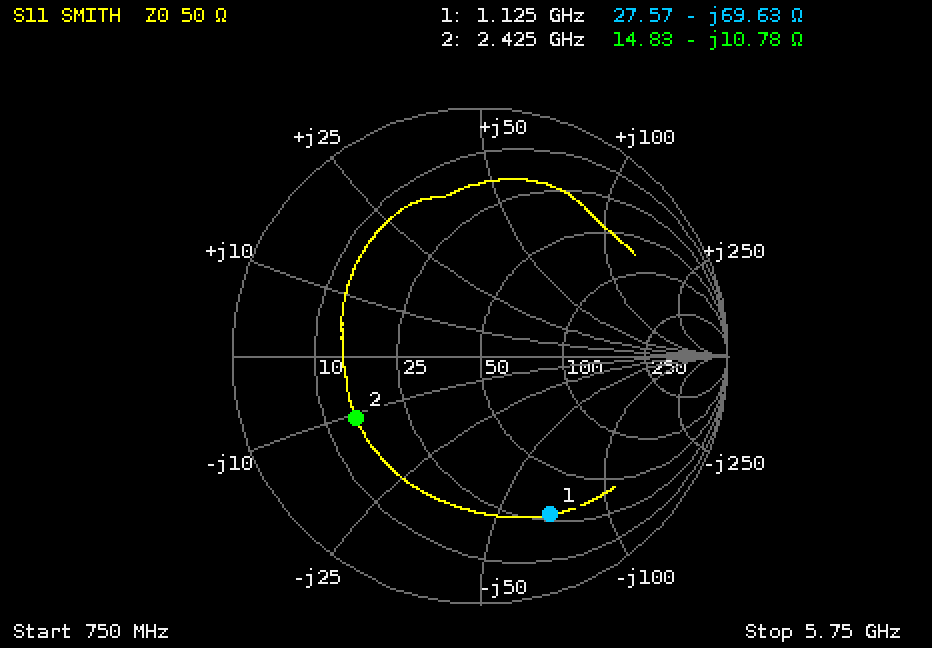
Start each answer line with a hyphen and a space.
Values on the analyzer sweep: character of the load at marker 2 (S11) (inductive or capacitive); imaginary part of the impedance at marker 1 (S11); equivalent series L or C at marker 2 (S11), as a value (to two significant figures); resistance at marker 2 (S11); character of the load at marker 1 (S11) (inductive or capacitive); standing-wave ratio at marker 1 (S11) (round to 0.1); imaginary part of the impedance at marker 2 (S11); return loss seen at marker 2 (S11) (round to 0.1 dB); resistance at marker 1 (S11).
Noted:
- capacitive
- -69.63 Ω
- 6.1 pF
- 14.83 Ω
- capacitive
- 5.7
- -10.78 Ω
- 5.0 dB
- 27.57 Ω
